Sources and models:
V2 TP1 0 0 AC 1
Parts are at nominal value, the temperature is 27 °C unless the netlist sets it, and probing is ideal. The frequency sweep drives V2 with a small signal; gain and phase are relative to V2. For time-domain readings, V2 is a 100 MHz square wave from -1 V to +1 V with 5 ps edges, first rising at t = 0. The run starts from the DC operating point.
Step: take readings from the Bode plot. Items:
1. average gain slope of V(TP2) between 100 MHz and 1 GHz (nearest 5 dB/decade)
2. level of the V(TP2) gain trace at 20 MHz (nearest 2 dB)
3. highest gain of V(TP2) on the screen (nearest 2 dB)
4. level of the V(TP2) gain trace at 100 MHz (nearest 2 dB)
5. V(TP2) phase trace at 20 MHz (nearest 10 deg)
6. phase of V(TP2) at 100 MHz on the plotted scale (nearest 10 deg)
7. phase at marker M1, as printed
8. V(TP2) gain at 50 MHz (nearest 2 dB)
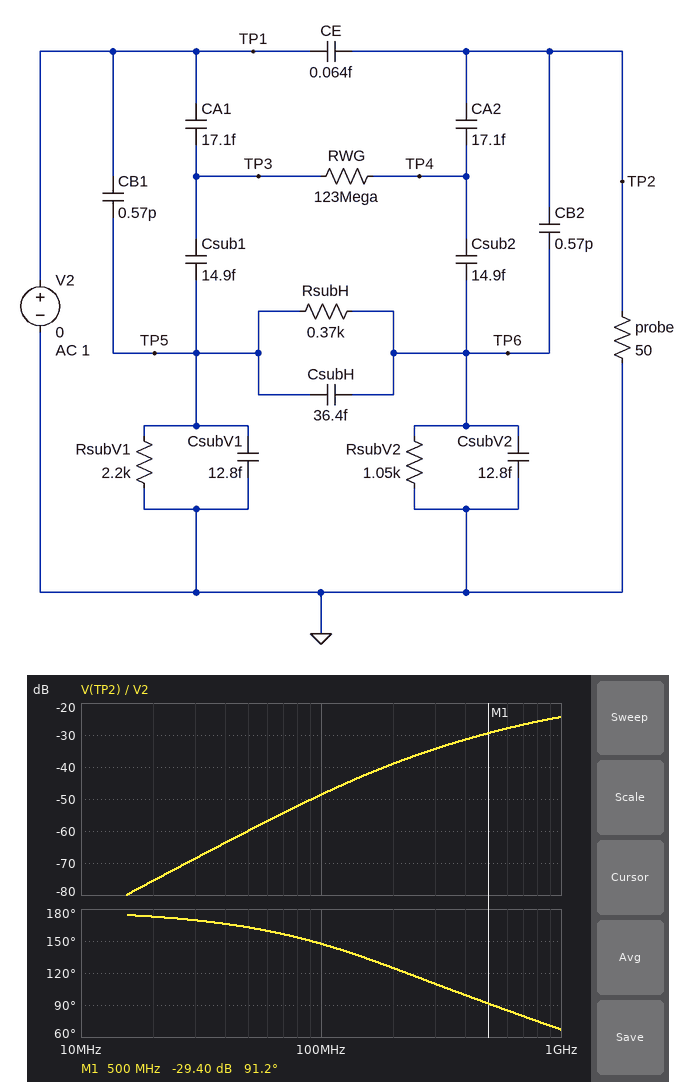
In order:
25 dB/decade
-76 dB
-24 dB
-48 dB
170 deg
150 deg
91.2 deg
-60 dB
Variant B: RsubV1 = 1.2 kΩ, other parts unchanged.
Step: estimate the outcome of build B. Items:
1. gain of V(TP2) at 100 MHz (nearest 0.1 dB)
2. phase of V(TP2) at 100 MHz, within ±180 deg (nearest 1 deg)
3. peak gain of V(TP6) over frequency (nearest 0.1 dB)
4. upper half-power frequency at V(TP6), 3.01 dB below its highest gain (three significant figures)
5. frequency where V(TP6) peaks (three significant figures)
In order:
-50.7 dB
153 deg
-9.1 dB
1.95 GHz
578 MHz
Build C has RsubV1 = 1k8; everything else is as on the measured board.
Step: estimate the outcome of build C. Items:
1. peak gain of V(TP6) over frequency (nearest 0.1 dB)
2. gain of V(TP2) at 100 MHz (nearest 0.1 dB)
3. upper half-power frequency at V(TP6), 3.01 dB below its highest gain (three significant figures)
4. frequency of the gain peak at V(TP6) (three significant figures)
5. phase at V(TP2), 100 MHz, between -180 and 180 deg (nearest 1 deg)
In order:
-8.7 dB
-49.3 dB
1.83 GHz
522 MHz
149 deg
